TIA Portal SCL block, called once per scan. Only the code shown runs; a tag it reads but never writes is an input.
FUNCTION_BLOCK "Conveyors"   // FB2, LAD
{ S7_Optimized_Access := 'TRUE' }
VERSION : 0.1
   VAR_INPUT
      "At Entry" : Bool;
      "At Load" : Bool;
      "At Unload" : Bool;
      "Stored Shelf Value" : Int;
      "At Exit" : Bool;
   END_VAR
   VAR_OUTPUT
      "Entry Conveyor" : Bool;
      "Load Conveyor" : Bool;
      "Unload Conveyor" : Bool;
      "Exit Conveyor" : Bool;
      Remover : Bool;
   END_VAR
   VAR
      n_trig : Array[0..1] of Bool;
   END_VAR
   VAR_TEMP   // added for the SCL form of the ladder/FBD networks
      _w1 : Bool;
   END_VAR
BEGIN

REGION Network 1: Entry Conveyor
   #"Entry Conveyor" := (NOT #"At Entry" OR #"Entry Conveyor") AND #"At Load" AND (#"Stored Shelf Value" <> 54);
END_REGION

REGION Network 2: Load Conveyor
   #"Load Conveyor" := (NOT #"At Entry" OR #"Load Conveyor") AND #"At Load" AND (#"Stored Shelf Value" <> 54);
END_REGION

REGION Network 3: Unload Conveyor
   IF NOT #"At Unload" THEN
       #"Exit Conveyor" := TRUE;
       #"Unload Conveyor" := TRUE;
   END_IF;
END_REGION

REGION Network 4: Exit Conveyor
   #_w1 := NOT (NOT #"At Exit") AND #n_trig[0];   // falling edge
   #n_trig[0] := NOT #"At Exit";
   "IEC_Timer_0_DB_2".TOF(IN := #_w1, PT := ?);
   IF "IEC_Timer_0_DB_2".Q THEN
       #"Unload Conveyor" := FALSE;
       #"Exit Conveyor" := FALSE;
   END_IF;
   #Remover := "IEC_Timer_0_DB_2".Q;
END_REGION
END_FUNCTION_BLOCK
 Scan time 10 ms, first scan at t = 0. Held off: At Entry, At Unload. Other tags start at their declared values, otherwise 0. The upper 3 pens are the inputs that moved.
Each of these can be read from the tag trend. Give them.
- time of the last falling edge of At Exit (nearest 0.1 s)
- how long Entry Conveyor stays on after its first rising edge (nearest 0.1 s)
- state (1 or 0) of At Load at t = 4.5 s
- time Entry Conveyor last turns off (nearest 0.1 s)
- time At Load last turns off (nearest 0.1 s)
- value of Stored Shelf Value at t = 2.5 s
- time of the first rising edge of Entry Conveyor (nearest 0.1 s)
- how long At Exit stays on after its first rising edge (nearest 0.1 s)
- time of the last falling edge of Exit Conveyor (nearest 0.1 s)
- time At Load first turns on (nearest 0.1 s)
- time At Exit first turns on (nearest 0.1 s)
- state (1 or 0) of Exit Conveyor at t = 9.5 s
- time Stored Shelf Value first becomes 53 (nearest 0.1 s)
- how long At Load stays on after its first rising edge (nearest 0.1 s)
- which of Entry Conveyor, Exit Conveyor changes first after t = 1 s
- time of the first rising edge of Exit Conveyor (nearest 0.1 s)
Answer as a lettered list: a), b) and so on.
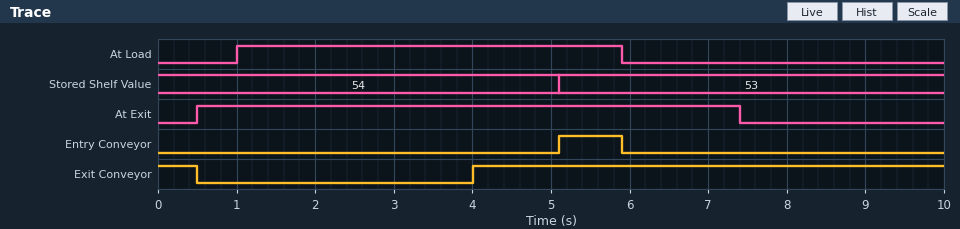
a) 7.4 s
b) 0.8 s
c) 1
d) 5.9 s
e) 5.9 s
f) 54
g) 5.1 s
h) 6.9 s
i) 0.5 s
j) 1.0 s
k) 0.5 s
l) 1
m) 5.1 s
n) 4.9 s
o) Exit Conveyor
p) 4.0 s
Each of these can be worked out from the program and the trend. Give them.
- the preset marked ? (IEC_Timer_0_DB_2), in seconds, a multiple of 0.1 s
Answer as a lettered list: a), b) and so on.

a) 3.5 s
